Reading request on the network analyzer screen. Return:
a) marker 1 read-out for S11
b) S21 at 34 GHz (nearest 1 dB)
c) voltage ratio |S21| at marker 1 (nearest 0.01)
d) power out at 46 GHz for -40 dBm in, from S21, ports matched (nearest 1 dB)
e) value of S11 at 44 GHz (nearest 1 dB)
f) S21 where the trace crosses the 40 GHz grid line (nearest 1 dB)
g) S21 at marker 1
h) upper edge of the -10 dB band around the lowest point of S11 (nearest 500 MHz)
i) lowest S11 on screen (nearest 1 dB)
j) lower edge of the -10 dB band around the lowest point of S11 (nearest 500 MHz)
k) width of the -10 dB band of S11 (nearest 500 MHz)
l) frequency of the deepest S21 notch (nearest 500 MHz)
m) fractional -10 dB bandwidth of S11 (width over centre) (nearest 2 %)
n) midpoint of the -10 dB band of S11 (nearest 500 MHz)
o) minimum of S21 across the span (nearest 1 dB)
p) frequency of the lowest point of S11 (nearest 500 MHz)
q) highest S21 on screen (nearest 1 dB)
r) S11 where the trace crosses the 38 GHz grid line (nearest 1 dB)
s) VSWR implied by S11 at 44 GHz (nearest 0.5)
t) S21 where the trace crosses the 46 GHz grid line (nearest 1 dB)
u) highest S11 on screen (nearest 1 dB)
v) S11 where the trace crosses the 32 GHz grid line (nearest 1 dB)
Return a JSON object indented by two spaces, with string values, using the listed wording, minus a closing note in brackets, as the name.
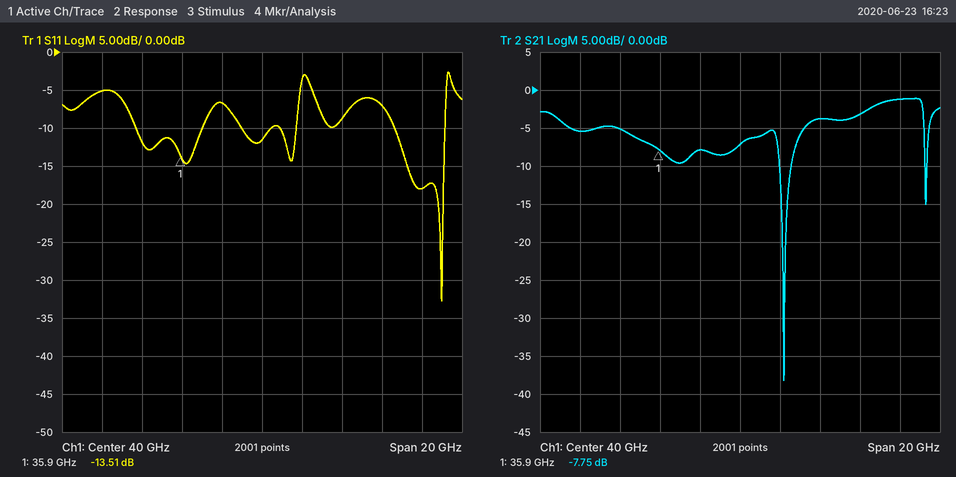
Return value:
{
  "marker 1 read-out for S11": "-13.51 dB",
  "S21 at 34 GHz": "-5 dB",
  "voltage ratio |S21| at marker 1": "0.41",
  "power out at 46 GHz for -40 dBm in, from S21, ports matched": "-43 dBm",
  "value of S11 at 44 GHz": "-9 dB",
  "S21 where the trace crosses the 40 GHz grid line": "-7 dB",
  "S21 at marker 1": "-7.75 dB",
  "upper edge of the -10 dB band around the lowest point of S11": "49.0 GHz",
  "lowest S11 on screen": "-33 dB",
  "lower edge of the -10 dB band around the lowest point of S11": "46.5 GHz",
  "width of the -10 dB band of S11": "2.5 GHz",
  "frequency of the deepest S21 notch": "42.0 GHz",
  "fractional -10 dB bandwidth of S11 (width over centre)": "6 %",
  "midpoint of the -10 dB band of S11": "48.0 GHz",
  "minimum of S21 across the span": "-38 dB",
  "frequency of the lowest point of S11": "49.0 GHz",
  "highest S21 on screen": "-1 dB",
  "S11 where the trace crosses the 38 GHz grid line": "-7 dB",
  "VSWR implied by S11 at 44 GHz": "2.0",
  "S21 where the trace crosses the 46 GHz grid line": "-3 dB",
  "highest S11 on screen": "-3 dB",
  "S11 where the trace crosses the 32 GHz grid line": "-5 dB"
}
